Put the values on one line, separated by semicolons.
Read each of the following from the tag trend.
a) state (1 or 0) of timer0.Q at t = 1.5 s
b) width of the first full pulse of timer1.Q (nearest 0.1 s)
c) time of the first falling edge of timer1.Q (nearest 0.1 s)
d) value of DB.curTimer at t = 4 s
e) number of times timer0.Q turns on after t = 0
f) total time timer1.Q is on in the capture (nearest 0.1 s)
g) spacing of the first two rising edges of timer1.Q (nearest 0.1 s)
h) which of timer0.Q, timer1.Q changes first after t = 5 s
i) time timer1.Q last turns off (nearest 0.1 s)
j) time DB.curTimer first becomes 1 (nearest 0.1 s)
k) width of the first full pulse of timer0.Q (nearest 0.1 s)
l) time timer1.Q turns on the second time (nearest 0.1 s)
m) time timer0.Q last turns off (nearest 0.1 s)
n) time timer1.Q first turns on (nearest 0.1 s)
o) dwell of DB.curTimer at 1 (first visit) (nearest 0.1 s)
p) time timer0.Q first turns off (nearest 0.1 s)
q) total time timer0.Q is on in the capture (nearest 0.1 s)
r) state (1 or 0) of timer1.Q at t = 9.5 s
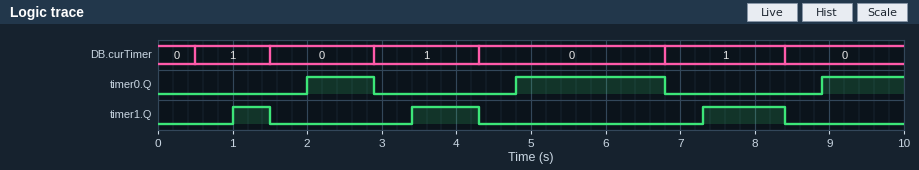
0; 0.5 s; 1.5 s; 1; 3; 2.5 s; 2.4 s; timer0.Q; 8.4 s; 0.5 s; 0.9 s; 3.4 s; 6.8 s; 1.0 s; 1.0 s; 2.9 s; 4.0 s; 0
